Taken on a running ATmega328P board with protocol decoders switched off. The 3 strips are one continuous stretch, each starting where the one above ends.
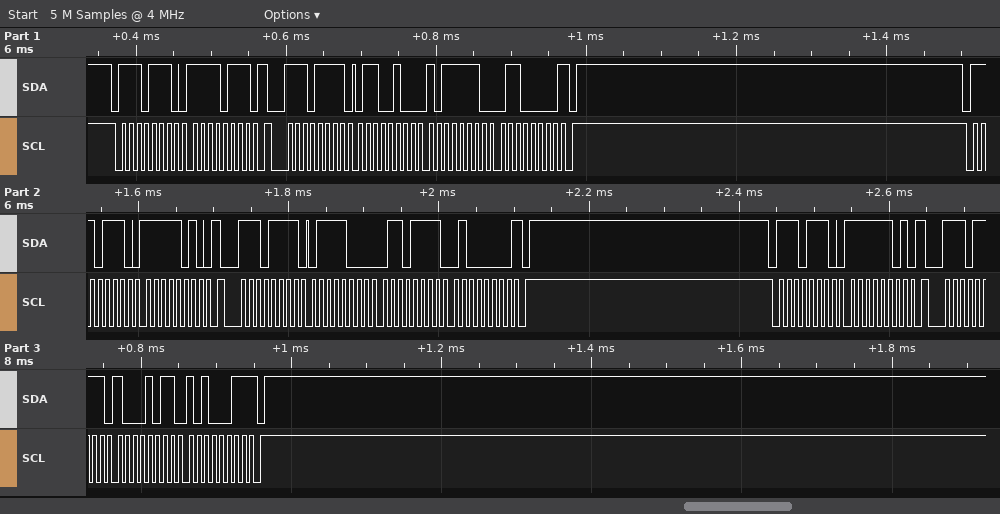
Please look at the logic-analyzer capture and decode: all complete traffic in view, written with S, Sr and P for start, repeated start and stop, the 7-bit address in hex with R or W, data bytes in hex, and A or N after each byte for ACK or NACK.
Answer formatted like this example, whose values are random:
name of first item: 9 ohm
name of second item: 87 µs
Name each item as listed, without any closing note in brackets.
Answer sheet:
all complete traffic in view, written with S, Sr and P for start, repeated start and stop, the 7-bit address in hex with R or W, data bytes in hex, and A or N after each byte for ACK or NACK: S 77W A F7 A Sr 77R A 64 A BE A 60 N P S 77W A FA A Sr 77R A 78 A 6F A 40 N P S 77W A FD A Sr 77R A 8B A A3 N P
